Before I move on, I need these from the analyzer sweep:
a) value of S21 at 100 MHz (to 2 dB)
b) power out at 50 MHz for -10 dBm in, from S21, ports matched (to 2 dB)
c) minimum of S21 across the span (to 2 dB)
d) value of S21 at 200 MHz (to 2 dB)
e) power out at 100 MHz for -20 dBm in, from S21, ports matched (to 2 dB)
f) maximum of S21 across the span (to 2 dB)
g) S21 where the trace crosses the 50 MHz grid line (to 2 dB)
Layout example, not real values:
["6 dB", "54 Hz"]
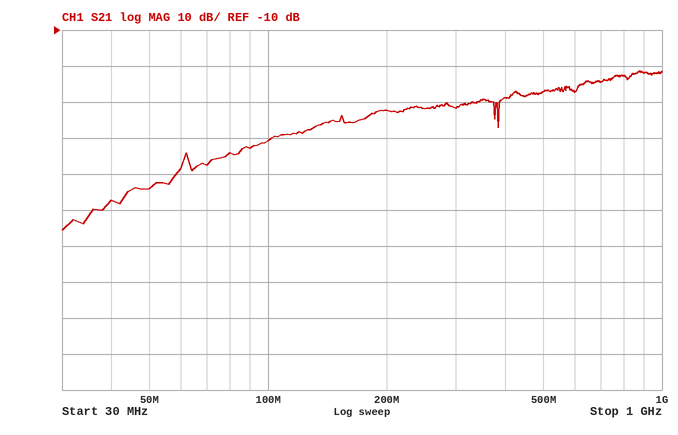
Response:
["-40 dB", "-64 dBm", "-66 dB", "-32 dB", "-60 dBm", "-22 dB", "-54 dB"]
